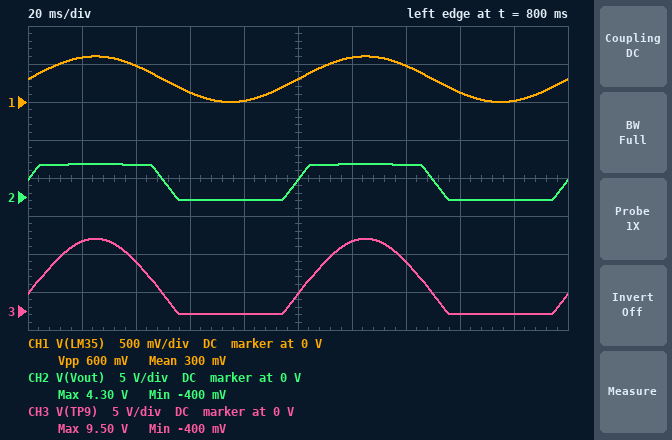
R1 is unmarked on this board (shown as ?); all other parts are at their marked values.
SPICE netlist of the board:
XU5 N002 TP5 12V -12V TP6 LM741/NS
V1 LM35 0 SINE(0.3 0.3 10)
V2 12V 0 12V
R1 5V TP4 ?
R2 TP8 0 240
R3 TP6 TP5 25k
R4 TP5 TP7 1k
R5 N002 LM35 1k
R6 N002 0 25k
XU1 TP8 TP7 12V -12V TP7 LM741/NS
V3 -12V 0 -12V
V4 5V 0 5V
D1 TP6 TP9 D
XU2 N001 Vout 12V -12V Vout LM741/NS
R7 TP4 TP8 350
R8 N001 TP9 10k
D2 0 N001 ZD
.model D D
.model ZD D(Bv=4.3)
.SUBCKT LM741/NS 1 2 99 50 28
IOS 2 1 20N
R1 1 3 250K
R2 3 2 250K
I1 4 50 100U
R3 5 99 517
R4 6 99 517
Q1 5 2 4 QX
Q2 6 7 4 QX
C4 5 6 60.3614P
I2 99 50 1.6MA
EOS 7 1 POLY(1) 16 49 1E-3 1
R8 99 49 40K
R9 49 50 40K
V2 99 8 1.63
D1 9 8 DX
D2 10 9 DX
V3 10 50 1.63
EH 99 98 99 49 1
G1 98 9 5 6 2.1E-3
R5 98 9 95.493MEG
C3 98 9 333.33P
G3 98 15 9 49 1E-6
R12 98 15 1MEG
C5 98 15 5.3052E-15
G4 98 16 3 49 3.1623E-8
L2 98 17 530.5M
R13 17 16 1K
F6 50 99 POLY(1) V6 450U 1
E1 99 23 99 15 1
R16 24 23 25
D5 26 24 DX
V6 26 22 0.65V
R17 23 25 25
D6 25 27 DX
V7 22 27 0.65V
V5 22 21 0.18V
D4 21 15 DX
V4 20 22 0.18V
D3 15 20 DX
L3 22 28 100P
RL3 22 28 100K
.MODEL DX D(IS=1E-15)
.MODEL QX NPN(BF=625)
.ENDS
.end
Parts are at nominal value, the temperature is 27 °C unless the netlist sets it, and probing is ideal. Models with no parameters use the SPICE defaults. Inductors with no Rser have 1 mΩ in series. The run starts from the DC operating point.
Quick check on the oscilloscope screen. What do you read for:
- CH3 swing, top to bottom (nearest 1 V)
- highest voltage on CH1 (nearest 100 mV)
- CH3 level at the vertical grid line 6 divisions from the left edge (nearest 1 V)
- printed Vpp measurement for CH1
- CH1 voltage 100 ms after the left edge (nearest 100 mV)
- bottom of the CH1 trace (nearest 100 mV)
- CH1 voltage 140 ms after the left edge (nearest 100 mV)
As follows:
10 V
600 mV
9 V
600 mV
300 mV
0 V
500 mV
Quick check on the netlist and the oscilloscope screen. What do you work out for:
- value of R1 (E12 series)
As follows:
5.6 kΩ
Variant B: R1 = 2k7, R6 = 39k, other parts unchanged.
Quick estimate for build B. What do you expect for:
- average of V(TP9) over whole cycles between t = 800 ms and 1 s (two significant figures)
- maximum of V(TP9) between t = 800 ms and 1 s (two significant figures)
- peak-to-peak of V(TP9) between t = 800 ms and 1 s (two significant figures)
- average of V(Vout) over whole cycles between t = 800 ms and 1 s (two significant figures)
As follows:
1.3 V
5.5 V
5.9 V
1.1 V
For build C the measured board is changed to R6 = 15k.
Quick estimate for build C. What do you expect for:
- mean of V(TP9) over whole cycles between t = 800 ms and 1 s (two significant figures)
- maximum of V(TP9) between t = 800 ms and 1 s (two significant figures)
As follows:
3.2 V
9.1 V
